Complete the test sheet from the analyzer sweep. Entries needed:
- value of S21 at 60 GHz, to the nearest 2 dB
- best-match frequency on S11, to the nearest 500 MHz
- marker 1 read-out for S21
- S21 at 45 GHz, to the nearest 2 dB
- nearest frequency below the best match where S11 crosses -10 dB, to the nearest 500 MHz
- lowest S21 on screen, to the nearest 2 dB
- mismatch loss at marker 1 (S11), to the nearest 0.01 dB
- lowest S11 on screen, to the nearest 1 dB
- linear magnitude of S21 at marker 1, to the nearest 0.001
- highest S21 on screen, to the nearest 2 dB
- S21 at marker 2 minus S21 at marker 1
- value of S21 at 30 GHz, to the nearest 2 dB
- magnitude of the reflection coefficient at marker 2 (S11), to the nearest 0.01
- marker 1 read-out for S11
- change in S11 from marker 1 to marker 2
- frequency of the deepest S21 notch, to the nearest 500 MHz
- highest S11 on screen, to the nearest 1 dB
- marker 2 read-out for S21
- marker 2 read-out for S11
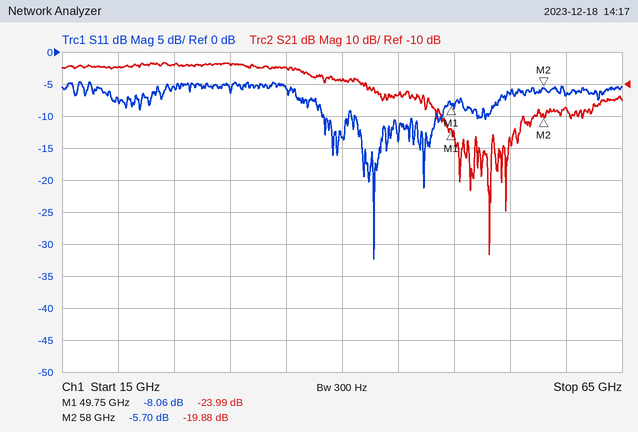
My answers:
-18 dB
43.0 GHz
-23.99 dB
-14 dB
41.0 GHz
-64 dB
0.74 dB
-32 dB
0.063
-4 dB
4.11 dB
-4 dB
0.52
-8.06 dB
2.36 dB
53.0 GHz
-5 dB
-19.88 dB
-5.70 dB
